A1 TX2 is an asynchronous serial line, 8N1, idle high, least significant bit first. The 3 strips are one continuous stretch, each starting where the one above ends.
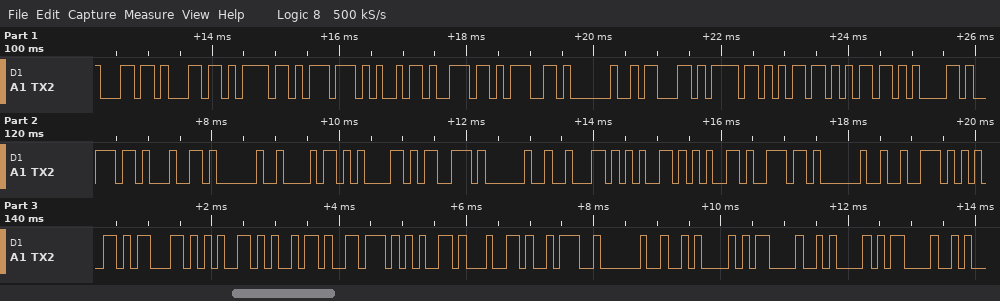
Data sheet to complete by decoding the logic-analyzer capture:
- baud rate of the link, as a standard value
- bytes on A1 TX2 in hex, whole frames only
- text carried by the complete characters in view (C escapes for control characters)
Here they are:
9600 baud
0x6C 0x6C 0x6F 0x77 0x69 0x6E 0x67 0x20 0x63 0x6F 0x6D 0x6D 0x61 0x6E 0x64 0x20 0x68 0x61 0x73 0x20 0x62 0x65 0x65 0x6E 0x20 0x72 0x65 0x63 0x65 0x69 0x76 0x65 0x64 0x3A 0x20 0x0A 0x0D 0x0A 0x0D
"llowing command has been received: \n\r\n\r"
